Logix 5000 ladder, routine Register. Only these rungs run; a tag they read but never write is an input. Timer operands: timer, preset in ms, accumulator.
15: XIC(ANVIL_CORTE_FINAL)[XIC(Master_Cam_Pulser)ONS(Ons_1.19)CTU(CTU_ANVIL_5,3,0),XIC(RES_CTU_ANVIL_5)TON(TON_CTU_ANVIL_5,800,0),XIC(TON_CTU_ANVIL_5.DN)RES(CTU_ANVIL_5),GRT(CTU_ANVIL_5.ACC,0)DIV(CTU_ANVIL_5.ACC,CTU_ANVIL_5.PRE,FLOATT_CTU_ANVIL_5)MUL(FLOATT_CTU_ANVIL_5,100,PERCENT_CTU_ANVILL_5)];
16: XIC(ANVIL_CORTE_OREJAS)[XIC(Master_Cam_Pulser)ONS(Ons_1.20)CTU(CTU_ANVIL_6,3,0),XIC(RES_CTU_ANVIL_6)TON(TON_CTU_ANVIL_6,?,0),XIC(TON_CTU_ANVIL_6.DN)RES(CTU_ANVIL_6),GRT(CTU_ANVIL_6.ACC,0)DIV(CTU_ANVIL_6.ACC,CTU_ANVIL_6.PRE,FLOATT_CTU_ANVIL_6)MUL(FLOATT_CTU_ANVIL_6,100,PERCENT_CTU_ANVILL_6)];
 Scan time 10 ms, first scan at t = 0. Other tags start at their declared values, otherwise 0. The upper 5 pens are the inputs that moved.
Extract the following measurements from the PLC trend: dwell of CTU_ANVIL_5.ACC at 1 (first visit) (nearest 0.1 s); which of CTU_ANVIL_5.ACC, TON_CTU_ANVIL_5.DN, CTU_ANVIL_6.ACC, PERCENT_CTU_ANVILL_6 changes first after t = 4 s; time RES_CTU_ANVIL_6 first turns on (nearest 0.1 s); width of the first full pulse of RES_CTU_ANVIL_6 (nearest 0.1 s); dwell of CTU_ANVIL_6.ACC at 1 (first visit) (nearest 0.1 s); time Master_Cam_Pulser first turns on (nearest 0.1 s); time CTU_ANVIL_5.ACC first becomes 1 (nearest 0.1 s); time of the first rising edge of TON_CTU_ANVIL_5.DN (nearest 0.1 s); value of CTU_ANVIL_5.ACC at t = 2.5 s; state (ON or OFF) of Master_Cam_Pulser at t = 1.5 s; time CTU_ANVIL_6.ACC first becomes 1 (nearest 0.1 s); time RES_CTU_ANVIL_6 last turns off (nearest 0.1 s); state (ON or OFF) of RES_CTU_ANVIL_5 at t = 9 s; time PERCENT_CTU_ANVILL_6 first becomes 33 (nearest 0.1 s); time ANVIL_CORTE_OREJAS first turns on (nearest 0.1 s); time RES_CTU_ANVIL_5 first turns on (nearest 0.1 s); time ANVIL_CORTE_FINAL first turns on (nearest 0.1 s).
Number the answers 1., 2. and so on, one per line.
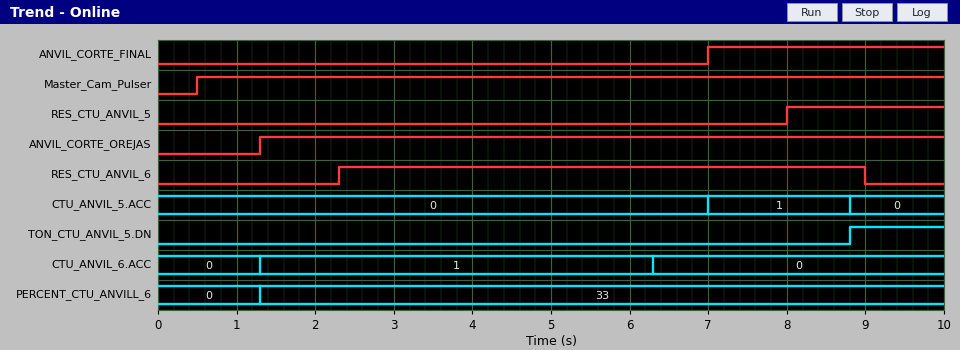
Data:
1. 1.8 s
2. CTU_ANVIL_6.ACC
3. 2.3 s
4. 6.7 s
5. 5.0 s
6. 0.5 s
7. 7.0 s
8. 8.8 s
9. 0
10. ON
11. 1.3 s
12. 9.0 s
13. ON
14. 1.3 s
15. 1.3 s
16. 8.0 s
17. 7.0 s
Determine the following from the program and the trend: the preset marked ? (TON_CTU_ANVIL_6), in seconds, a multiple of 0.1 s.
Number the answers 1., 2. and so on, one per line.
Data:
1. 4.0 s
